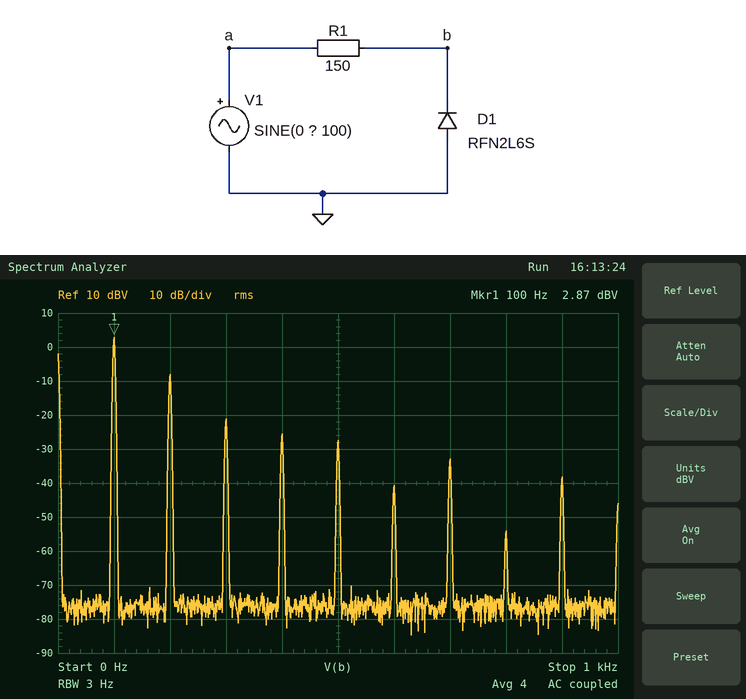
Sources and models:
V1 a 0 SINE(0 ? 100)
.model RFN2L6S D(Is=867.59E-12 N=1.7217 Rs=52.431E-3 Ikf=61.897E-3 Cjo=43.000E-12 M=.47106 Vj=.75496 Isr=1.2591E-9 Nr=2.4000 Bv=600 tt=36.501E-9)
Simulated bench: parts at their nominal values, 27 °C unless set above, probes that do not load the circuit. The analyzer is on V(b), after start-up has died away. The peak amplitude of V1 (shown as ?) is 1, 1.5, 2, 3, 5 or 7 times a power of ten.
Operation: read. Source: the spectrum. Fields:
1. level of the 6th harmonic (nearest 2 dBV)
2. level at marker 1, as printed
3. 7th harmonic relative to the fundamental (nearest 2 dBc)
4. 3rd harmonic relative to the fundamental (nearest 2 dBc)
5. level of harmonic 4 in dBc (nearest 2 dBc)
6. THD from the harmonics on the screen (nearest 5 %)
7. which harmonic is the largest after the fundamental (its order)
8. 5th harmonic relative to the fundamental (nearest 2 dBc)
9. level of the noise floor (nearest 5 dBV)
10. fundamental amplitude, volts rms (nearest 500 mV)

-40 dBV
2.87 dBV
-36 dBc
-24 dBc
-28 dBc
30 %
2
-30 dBc
-75 dBV
1.5 V
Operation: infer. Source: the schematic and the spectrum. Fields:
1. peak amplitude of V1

3 V
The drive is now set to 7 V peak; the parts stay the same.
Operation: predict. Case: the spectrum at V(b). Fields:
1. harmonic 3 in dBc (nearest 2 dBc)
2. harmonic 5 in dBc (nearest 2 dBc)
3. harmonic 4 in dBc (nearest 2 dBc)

-28 dBc
-34 dBc
-24 dBc
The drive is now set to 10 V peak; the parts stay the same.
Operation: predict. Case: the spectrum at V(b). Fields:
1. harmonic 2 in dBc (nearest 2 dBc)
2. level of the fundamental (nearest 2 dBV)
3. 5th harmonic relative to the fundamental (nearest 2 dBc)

-8 dBc
12 dBV
-36 dBc
